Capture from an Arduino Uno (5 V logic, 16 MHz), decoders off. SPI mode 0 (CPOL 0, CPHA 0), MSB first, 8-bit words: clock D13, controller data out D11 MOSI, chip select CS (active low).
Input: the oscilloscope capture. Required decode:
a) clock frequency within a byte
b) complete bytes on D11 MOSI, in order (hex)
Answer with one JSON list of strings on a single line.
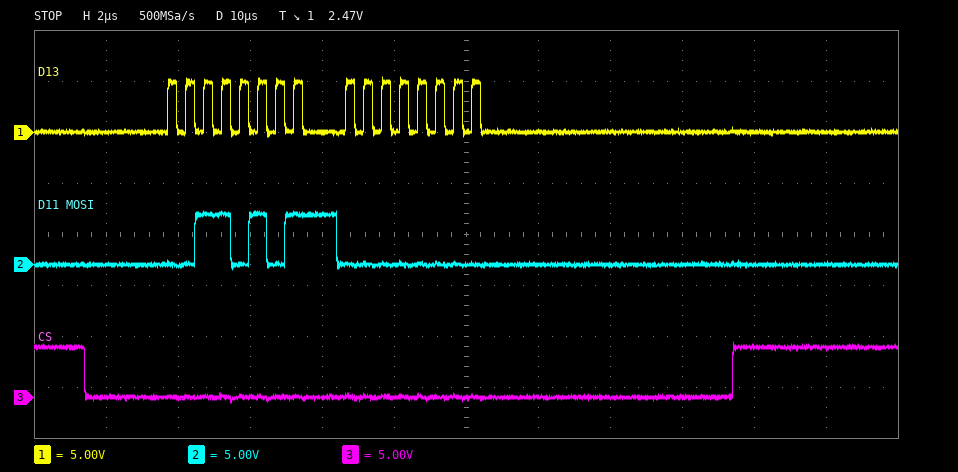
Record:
["2 MHz", "35 00"]
